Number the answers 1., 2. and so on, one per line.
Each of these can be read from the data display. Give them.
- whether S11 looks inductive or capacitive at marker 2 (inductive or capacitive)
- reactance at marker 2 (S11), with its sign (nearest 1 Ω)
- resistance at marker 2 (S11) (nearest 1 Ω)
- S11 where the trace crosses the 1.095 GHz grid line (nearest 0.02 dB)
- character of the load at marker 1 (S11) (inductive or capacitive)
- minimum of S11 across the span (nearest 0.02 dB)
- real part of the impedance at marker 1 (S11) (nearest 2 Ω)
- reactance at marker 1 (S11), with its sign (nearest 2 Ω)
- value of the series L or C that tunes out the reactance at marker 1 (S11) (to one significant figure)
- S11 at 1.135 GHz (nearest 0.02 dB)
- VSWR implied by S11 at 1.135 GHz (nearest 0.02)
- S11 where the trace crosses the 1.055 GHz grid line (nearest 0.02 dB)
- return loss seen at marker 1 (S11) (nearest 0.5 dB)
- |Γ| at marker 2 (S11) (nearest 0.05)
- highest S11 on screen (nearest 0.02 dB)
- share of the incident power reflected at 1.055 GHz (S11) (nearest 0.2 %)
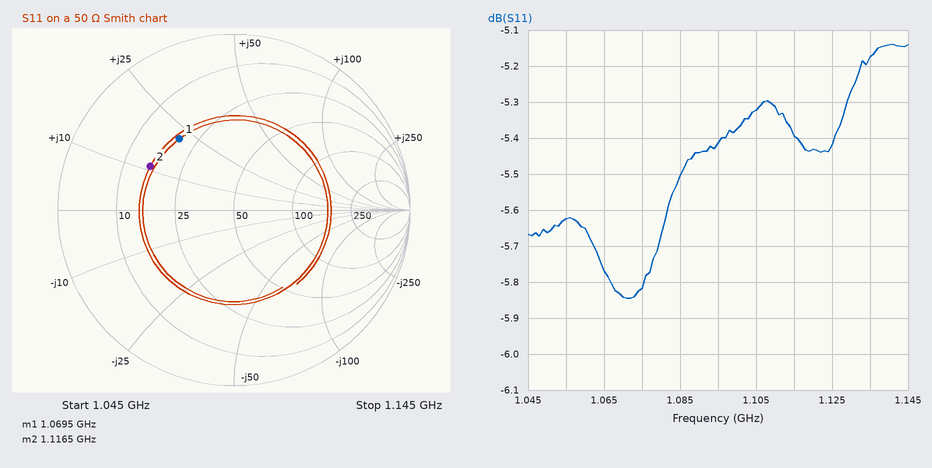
1. inductive
2. +11 Ω
3. 16 Ω
4. -5.42 dB
5. inductive
6. -5.84 dB
7. 20 Ω
8. +22 Ω
9. 7 pF
10. -5.18 dB
11. 3.46
12. -5.62 dB
13. 6.0 dB
14. 0.55
15. -5.14 dB
16. 27.4 %
